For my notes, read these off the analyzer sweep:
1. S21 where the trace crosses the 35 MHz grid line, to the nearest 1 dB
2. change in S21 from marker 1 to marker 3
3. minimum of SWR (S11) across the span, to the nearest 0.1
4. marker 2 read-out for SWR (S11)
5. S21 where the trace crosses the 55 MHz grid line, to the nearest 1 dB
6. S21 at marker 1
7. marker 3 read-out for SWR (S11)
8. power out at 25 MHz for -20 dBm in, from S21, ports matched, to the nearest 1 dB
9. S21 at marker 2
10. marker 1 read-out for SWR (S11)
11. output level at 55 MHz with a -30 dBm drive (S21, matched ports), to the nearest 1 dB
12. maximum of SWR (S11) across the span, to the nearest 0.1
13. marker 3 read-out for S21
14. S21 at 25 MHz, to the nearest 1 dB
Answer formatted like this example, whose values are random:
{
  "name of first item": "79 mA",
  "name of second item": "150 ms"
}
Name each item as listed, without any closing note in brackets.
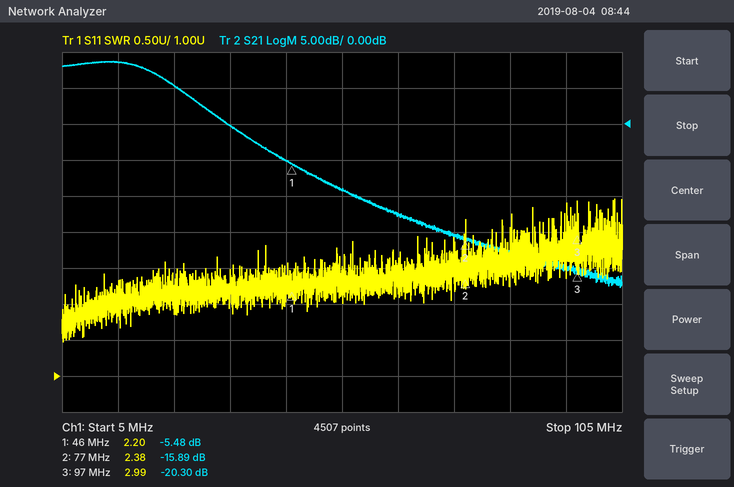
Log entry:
{
  "S21 where the trace crosses the 35 MHz grid line, to the nearest 1 dB": "0 dB",
  "change in S21 from marker 1 to marker 3": "-14.82 dB",
  "minimum of SWR (S11) across the span, to the nearest 0.1": "1.5",
  "marker 2 read-out for SWR": "2.38",
  "S21 where the trace crosses the 55 MHz grid line, to the nearest 1 dB": "-9 dB",
  "S21 at marker 1": "-5.48 dB",
  "marker 3 read-out for SWR": "2.99",
  "power out at 25 MHz for -20 dBm in, from S21, ports matched, to the nearest 1 dB": "-15 dBm",
  "S21 at marker 2": "-15.89 dB",
  "marker 1 read-out for SWR": "2.20",
  "output level at 55 MHz with a -30 dBm drive (S21, matched ports), to the nearest 1 dB": "-39 dBm",
  "maximum of SWR (S11) across the span, to the nearest 0.1": "3.5",
  "marker 3 read-out for S21": "-20.30 dB",
  "S21 at 25 MHz, to the nearest 1 dB": "5 dB"
}
